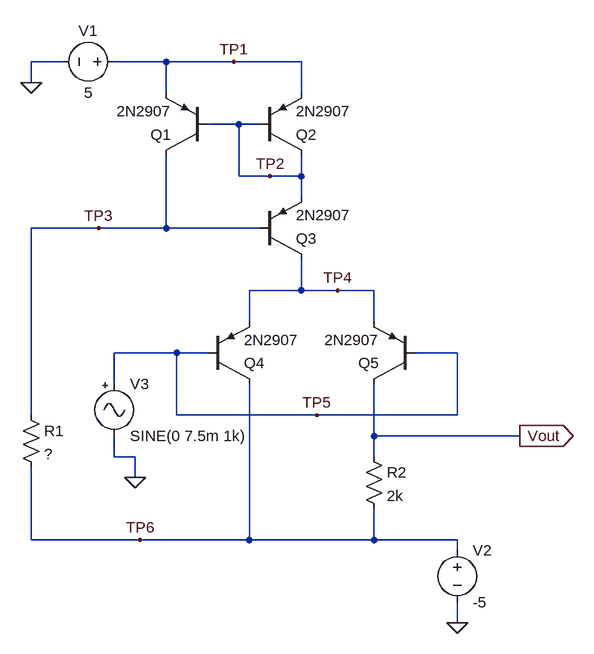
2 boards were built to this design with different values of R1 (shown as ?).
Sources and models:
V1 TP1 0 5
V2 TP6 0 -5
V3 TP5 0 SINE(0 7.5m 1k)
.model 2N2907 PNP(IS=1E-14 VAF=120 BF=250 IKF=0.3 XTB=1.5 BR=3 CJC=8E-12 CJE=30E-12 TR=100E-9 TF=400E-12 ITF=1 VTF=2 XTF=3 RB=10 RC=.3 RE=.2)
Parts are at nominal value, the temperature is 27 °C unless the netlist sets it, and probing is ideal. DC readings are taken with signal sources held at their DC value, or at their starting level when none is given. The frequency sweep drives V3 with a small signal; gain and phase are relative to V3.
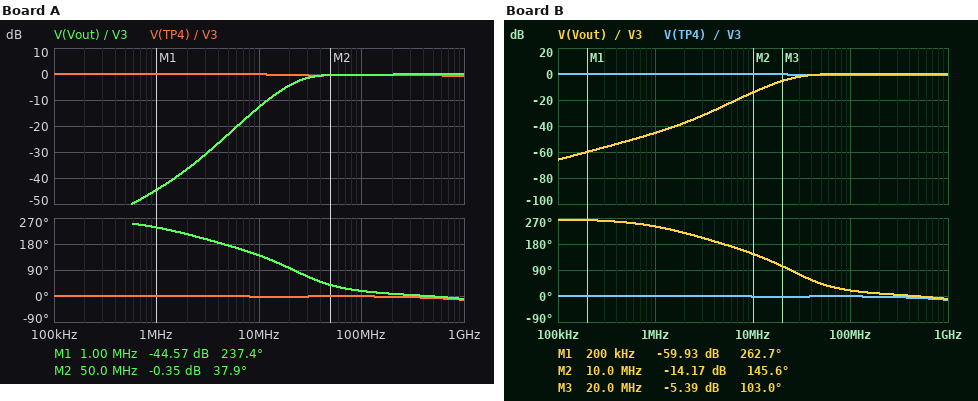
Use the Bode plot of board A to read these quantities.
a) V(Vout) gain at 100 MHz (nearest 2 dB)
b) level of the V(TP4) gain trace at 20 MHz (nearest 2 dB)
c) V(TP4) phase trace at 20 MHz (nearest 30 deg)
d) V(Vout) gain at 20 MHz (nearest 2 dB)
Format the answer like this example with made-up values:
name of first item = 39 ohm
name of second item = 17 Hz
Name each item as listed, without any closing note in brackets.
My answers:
V(Vout) gain at 100 MHz = 0 dB
level of the V(TP4) gain trace at 20 MHz = 0 dB
V(TP4) phase trace at 20 MHz = 0 deg
V(Vout) gain at 20 MHz = -4 dB
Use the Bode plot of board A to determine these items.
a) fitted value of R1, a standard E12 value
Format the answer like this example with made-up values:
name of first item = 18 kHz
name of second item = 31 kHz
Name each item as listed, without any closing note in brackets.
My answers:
fitted value of R1, a standard E12 value = 22 kΩ
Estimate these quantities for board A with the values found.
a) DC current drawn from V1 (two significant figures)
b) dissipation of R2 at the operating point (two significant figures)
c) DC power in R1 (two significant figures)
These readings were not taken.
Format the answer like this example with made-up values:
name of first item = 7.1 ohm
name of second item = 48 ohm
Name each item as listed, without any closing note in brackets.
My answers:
DC current drawn from V1 = 790 µA
dissipation of R2 at the operating point = 77 µW
DC power in R1 = 3.5 mW
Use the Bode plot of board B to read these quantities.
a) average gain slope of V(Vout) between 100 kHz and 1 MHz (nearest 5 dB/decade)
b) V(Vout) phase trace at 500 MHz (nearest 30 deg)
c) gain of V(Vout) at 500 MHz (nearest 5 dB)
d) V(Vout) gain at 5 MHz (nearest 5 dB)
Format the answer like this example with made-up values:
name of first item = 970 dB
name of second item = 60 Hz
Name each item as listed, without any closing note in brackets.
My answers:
average gain slope of V(Vout) between 100 kHz and 1 MHz = 20 dB/decade
V(Vout) phase trace at 500 MHz = 0 deg
gain of V(Vout) at 500 MHz = 0 dB
V(Vout) gain at 5 MHz = -25 dB
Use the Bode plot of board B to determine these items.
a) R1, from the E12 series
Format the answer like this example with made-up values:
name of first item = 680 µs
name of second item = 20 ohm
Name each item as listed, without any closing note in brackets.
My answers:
R1, from the E12 series = 18 kΩ
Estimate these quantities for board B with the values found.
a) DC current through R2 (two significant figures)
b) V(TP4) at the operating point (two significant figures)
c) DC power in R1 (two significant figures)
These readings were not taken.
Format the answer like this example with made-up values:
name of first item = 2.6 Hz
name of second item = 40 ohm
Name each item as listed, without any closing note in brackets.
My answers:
DC current through R2 = 240 µA
V(TP4) at the operating point = 620 mV
DC power in R1 = 4.2 mW
